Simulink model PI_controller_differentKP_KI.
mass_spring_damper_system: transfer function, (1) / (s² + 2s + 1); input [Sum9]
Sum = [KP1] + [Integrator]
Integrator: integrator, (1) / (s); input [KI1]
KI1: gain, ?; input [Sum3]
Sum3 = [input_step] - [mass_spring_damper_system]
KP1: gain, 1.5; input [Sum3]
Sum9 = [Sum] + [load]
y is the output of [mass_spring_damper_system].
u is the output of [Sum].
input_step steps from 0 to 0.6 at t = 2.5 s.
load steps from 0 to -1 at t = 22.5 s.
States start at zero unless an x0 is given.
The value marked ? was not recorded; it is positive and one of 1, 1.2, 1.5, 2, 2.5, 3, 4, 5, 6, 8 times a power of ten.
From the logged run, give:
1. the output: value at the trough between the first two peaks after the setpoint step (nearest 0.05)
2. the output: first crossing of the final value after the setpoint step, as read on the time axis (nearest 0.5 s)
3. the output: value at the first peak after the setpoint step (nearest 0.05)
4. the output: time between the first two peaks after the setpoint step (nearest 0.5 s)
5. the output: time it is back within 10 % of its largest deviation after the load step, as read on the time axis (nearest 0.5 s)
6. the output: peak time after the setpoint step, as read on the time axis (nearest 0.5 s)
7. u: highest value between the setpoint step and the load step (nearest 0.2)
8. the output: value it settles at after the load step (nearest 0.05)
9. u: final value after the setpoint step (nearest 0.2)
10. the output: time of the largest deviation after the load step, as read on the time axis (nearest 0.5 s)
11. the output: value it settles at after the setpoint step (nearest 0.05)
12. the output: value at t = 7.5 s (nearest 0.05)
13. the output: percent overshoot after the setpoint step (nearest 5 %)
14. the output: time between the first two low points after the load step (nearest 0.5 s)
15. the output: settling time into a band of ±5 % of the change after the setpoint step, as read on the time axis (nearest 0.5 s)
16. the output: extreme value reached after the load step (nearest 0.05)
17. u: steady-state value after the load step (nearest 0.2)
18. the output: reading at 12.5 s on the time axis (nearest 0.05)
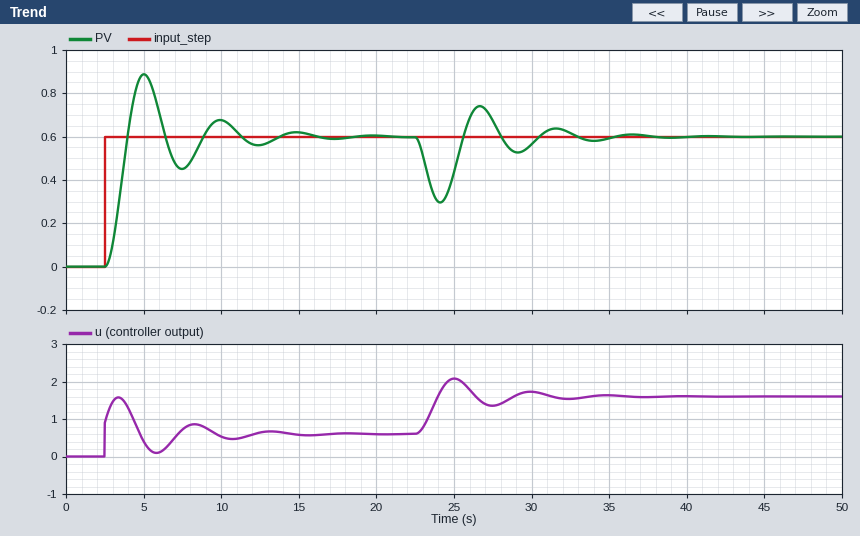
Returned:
0.45
4.0 s
0.90
5.0 s
32.0 s
5.0 s
1.6
0.60
0.6
24.0 s
0.60
0.45
50 %
5.0 s
13.0 s
0.30
1.6
0.55
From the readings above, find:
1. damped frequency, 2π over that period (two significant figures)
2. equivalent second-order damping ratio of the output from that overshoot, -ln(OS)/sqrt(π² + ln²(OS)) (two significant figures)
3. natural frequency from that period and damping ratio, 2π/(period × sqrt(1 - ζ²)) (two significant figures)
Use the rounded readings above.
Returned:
1.3 rad/s
0.22
1.3 rad/s
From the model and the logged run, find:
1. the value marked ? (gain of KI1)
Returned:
2.5
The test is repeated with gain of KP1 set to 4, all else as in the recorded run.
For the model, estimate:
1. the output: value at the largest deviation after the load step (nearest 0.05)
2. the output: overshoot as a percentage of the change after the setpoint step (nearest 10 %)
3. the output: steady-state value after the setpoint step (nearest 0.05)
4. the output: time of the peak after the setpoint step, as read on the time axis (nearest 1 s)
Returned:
0.40
30 %
0.60
4 s
